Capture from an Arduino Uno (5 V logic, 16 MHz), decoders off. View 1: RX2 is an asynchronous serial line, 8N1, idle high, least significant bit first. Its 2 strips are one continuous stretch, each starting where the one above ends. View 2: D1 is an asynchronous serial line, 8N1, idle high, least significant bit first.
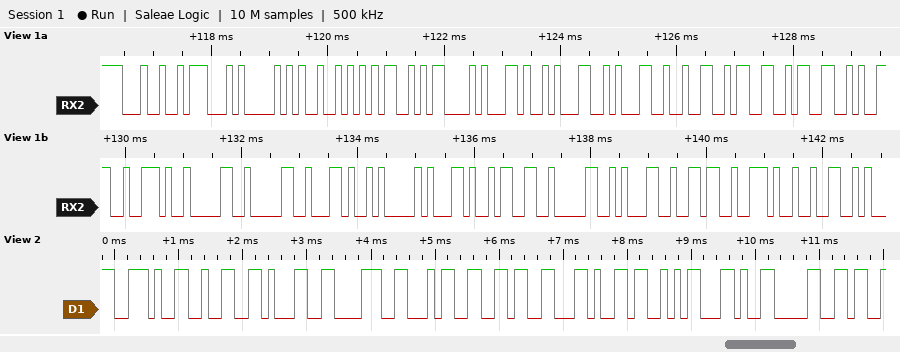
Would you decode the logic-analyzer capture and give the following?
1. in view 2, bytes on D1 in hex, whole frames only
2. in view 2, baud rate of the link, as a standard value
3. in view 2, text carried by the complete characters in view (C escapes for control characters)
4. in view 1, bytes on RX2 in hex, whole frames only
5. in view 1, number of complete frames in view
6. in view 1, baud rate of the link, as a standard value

2E 32 31 38 34 36 2C 53 2C 30
9600 baud
".21846,S,0"
24 47 50 52 4D 43 2C 31 31 32 33 33 39 2E 30 30 2C 41 2C 33 30 31 36 2E 32
25
9600 baud
